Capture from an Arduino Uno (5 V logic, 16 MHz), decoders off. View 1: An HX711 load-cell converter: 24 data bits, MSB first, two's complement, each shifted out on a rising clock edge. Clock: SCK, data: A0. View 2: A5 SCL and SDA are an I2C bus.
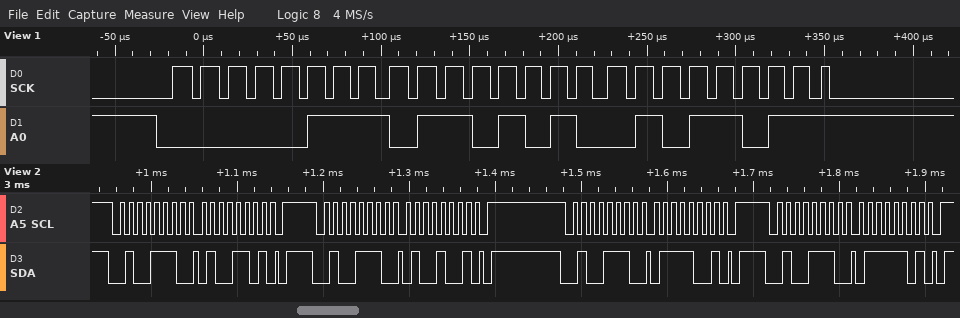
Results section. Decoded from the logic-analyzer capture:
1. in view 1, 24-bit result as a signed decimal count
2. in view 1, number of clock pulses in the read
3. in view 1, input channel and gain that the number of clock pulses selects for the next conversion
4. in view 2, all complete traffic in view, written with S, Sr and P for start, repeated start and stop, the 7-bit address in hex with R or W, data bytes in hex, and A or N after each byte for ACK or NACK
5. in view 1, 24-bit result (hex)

485979
25
channel A, gain 128
S 27W A 4D A P S 27W A 49 A P S 27W A 79 A P S 27W A 7D A P
0x076A5B
